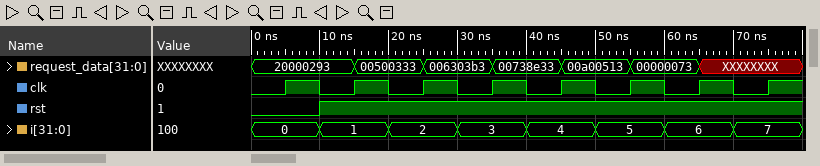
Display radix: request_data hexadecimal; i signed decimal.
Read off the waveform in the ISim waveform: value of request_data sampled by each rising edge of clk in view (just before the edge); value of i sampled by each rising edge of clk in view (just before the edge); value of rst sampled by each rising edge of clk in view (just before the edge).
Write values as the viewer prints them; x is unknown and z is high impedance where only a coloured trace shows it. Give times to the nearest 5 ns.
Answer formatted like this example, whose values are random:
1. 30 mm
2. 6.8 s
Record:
1. 20000293, 20000293, 00500333, 006303b3, 00738e33, 00a00513, 00000073, XXXXXXXX
2. 0, 1, 2, 3, 4, 5, 6, 7
3. 0 1 1 1 1 1 1 1
